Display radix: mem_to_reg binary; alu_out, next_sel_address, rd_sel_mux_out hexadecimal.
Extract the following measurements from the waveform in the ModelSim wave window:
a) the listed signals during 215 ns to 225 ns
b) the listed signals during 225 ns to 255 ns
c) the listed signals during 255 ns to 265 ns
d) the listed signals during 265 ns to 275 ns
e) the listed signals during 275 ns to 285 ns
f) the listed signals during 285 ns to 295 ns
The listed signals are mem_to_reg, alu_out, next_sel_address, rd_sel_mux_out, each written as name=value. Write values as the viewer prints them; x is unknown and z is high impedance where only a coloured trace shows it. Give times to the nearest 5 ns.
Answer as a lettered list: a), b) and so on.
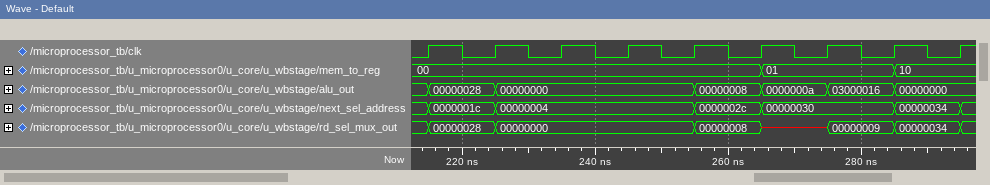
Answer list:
a) mem_to_reg=00, alu_out=00000028, next_sel_address=0000001c, rd_sel_mux_out=00000028
b) mem_to_reg=00, alu_out=00000000, next_sel_address=00000004, rd_sel_mux_out=00000000
c) mem_to_reg=00, alu_out=00000008, next_sel_address=0000002c, rd_sel_mux_out=00000008
d) mem_to_reg=01, alu_out=0000000a, next_sel_address=00000030, rd_sel_mux_out=x
e) mem_to_reg=01, alu_out=03000016, next_sel_address=00000030, rd_sel_mux_out=00000009
f) mem_to_reg=10, alu_out=00000000, next_sel_address=00000034, rd_sel_mux_out=00000034
